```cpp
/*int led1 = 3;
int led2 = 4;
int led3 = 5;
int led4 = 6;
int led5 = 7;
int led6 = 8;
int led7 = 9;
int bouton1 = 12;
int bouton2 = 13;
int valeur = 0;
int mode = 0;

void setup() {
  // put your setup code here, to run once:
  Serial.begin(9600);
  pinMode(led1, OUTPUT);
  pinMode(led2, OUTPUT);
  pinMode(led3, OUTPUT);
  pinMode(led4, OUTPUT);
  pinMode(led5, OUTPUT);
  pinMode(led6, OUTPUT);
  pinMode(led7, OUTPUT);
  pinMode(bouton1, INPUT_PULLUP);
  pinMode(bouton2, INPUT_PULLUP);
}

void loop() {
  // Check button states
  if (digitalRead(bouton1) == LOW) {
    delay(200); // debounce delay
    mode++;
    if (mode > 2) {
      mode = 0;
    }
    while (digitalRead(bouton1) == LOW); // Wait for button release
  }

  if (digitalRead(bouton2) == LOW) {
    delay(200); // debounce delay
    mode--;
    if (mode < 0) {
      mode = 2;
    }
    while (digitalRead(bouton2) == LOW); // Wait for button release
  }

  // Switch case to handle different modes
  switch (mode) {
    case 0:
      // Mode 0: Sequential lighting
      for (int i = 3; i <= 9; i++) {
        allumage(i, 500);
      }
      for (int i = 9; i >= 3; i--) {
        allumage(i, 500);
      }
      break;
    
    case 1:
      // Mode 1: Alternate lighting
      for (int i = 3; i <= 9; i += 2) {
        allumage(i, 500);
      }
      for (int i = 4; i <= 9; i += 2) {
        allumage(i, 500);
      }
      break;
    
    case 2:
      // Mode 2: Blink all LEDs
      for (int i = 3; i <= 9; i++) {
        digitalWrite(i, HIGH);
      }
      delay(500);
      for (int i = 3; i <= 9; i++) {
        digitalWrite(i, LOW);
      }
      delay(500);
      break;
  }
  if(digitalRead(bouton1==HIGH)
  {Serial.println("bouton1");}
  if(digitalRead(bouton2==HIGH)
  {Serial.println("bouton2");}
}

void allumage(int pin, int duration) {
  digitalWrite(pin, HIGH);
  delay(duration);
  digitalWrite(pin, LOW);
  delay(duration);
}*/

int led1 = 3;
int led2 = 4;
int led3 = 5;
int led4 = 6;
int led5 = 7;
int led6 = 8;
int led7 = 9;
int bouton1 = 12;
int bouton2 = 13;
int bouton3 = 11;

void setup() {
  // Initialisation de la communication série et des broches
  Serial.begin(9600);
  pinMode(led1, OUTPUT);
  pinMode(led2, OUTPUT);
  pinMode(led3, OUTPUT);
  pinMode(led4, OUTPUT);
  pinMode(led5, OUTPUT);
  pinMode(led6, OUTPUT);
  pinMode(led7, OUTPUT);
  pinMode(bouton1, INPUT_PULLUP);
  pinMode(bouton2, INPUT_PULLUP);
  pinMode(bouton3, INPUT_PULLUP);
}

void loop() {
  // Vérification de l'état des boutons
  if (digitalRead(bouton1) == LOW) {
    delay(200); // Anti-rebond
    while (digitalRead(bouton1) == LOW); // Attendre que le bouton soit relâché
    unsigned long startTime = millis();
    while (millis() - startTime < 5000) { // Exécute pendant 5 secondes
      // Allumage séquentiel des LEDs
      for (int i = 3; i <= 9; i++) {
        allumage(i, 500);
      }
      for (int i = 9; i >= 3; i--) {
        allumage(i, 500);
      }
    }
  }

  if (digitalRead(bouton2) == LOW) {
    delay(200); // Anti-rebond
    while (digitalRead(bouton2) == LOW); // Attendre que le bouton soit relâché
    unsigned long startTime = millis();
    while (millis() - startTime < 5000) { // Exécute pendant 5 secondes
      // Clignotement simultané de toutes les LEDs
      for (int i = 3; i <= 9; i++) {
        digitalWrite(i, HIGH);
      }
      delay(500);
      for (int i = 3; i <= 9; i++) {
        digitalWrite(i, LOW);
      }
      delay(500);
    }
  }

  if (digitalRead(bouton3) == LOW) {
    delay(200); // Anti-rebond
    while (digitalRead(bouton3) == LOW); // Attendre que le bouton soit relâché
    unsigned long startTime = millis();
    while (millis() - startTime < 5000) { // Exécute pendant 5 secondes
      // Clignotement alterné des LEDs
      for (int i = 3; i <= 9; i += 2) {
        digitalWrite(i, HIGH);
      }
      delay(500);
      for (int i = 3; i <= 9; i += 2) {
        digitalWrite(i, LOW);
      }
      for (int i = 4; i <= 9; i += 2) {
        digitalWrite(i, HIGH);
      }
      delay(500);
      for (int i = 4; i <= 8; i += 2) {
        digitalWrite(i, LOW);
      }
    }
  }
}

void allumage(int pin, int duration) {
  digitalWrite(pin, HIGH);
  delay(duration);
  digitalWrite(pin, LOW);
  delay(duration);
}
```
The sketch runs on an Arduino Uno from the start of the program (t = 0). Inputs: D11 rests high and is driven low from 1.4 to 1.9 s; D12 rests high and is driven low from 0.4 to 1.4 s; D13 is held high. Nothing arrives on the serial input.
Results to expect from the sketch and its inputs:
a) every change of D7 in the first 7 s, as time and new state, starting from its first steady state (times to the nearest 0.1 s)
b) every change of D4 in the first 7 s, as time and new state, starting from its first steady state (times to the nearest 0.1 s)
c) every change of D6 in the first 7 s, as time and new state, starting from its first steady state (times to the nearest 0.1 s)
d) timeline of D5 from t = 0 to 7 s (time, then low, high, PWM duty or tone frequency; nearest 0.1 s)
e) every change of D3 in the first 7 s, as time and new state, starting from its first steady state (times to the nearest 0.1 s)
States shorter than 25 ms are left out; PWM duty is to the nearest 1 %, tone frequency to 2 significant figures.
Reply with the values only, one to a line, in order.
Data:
0 s low; 5.4 s high; 5.9 s low
0 s low; 2.4 s high; 2.9 s low
0 s low; 4.4 s high; 4.9 s low
0 s low; 3.4 s high; 3.9 s low
0 s low; 1.4 s high; 1.9 s low
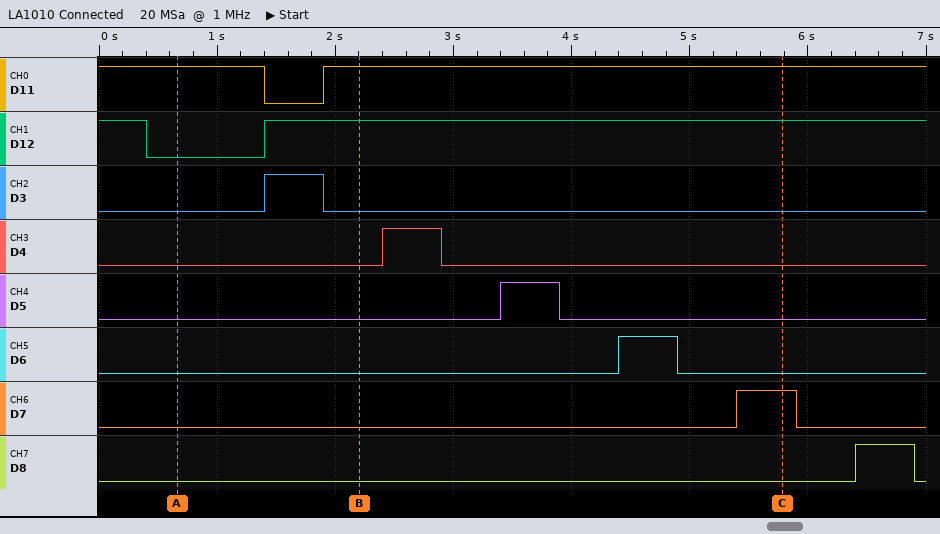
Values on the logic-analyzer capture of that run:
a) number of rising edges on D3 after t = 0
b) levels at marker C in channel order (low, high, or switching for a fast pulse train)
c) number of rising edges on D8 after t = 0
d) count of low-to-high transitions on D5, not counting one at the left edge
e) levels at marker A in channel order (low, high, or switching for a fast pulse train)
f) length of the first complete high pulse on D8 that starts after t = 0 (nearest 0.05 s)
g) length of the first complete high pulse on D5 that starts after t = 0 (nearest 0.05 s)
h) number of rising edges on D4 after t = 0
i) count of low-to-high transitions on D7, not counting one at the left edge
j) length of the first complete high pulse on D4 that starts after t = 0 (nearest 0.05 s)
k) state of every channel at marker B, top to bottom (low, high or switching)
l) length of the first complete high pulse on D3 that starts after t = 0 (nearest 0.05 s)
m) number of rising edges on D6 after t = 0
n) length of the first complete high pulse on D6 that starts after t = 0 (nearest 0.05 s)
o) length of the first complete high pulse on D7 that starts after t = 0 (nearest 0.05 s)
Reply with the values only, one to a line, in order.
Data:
1
D11 high, D12 high, D3 low, D4 low, D5 low, D6 low, D7 high, D8 low
1
1
D11 high, D12 low, D3 low, D4 low, D5 low, D6 low, D7 low, D8 low
0.50 s
0.50 s
1
1
0.50 s
D11 high, D12 high, D3 low, D4 low, D5 low, D6 low, D7 low, D8 low
0.50 s
1
0.50 s
0.50 s
